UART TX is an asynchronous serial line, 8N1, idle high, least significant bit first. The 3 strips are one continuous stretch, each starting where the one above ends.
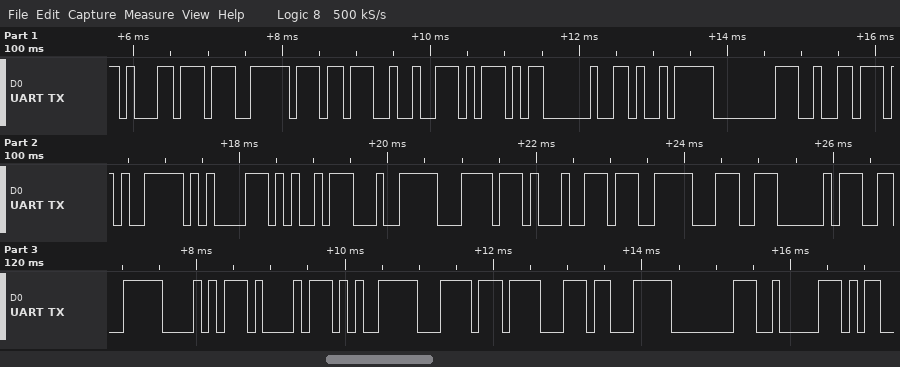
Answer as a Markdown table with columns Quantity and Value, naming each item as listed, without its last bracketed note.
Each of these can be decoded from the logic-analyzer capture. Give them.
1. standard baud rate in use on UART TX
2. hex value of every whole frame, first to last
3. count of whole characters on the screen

| Quantity | Value |
|---|---|
| standard baud rate in use on UART TX | 9600 baud |
| hex value of every whole frame, first to last | 0xB1 0xE7 0xB7 0x92 0x5D 0x20 0xE9 0x80 0xB2 0xE5 0x85 0xA5 0xE4 0xBC 0x91 0xE7 0x9C 0xA0 0xE6 0xA8 0xA1 0xE5 0xBC 0x8F 0xE3 0x80 0x82 |
| count of whole characters on the screen | 27 |
